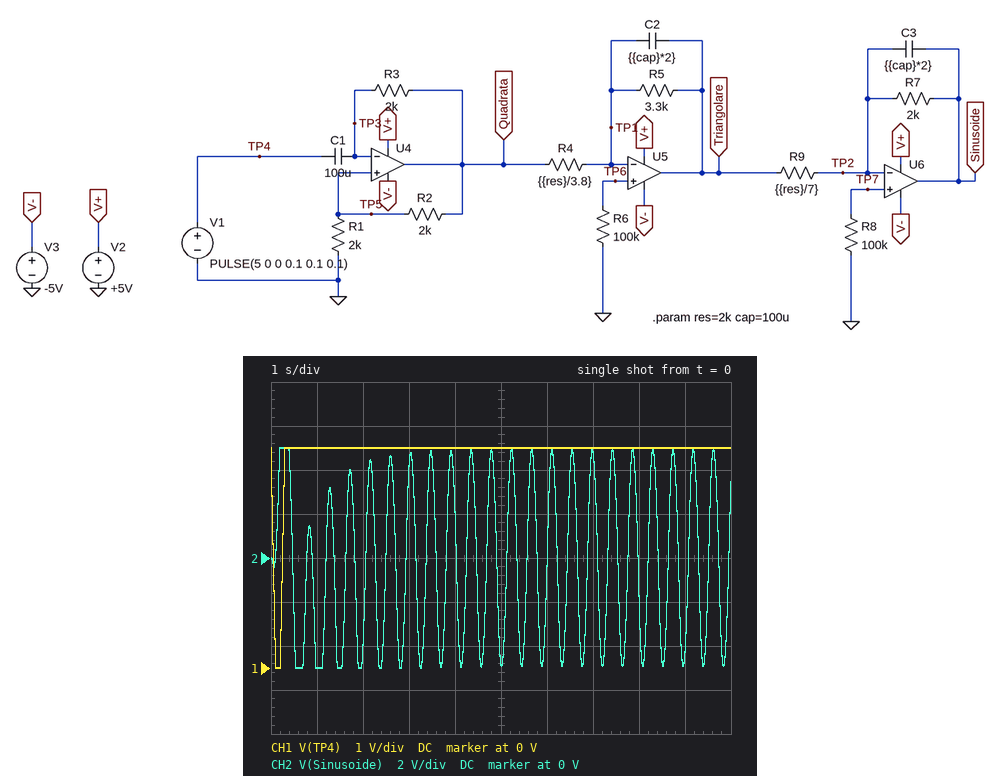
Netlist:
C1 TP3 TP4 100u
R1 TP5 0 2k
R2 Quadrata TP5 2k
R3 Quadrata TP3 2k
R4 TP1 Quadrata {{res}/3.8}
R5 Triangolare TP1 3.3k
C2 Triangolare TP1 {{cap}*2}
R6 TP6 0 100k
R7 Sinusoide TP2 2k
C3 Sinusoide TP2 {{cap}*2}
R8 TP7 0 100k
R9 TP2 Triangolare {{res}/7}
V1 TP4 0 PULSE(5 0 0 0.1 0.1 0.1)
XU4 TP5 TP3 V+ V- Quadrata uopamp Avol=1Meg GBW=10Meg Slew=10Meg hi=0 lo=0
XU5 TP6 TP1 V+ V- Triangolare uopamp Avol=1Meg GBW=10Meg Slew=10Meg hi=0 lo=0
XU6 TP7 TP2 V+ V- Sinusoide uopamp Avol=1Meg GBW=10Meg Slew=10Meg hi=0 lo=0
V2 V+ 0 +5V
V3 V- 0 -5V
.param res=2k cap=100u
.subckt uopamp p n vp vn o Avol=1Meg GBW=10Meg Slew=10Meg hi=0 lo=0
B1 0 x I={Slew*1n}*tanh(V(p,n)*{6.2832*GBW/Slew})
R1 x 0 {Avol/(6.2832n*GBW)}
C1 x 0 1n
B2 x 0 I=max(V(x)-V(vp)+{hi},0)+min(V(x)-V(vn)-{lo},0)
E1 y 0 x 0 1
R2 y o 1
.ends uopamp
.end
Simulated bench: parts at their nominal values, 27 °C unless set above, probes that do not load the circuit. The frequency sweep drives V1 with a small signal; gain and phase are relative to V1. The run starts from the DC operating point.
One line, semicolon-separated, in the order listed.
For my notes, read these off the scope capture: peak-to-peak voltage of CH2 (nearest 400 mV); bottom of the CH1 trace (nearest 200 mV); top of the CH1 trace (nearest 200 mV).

10.0 V; 0 V; 5.0 V
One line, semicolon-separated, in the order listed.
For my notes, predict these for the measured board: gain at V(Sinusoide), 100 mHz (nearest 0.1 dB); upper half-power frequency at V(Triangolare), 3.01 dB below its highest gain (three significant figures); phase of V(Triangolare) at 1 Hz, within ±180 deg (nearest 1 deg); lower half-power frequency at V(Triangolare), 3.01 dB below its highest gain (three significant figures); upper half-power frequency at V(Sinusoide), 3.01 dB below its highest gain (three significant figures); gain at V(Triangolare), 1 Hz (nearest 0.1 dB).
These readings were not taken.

19.8 dB; 1.20 Hz; 65 deg; 160 mHz; 594 mHz; 7.2 dB
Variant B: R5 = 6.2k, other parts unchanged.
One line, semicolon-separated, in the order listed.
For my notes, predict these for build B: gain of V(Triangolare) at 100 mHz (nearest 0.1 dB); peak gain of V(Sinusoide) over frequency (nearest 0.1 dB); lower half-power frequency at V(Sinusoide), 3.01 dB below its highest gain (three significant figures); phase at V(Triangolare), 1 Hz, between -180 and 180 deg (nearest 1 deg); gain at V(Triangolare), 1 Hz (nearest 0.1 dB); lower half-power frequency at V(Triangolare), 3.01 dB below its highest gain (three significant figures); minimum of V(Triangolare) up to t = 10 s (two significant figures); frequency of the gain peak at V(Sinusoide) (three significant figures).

7.3 dB; 25.8 dB; 80.0 mHz; 59 deg; 7.4 dB; 99.8 mHz; -5.0 V; 207 mHz
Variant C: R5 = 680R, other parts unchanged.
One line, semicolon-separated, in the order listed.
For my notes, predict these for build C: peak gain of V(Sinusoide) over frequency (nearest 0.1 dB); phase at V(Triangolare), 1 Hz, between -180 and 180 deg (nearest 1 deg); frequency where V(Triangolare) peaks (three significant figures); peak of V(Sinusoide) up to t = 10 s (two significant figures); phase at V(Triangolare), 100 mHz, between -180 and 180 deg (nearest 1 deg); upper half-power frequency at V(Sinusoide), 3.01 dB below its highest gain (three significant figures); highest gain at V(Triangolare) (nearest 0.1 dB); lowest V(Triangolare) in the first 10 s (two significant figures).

14.8 dB; 101 deg; 965 mHz; 5.0 V; 92 deg; 1.02 Hz; 3.7 dB; -4.6 V
